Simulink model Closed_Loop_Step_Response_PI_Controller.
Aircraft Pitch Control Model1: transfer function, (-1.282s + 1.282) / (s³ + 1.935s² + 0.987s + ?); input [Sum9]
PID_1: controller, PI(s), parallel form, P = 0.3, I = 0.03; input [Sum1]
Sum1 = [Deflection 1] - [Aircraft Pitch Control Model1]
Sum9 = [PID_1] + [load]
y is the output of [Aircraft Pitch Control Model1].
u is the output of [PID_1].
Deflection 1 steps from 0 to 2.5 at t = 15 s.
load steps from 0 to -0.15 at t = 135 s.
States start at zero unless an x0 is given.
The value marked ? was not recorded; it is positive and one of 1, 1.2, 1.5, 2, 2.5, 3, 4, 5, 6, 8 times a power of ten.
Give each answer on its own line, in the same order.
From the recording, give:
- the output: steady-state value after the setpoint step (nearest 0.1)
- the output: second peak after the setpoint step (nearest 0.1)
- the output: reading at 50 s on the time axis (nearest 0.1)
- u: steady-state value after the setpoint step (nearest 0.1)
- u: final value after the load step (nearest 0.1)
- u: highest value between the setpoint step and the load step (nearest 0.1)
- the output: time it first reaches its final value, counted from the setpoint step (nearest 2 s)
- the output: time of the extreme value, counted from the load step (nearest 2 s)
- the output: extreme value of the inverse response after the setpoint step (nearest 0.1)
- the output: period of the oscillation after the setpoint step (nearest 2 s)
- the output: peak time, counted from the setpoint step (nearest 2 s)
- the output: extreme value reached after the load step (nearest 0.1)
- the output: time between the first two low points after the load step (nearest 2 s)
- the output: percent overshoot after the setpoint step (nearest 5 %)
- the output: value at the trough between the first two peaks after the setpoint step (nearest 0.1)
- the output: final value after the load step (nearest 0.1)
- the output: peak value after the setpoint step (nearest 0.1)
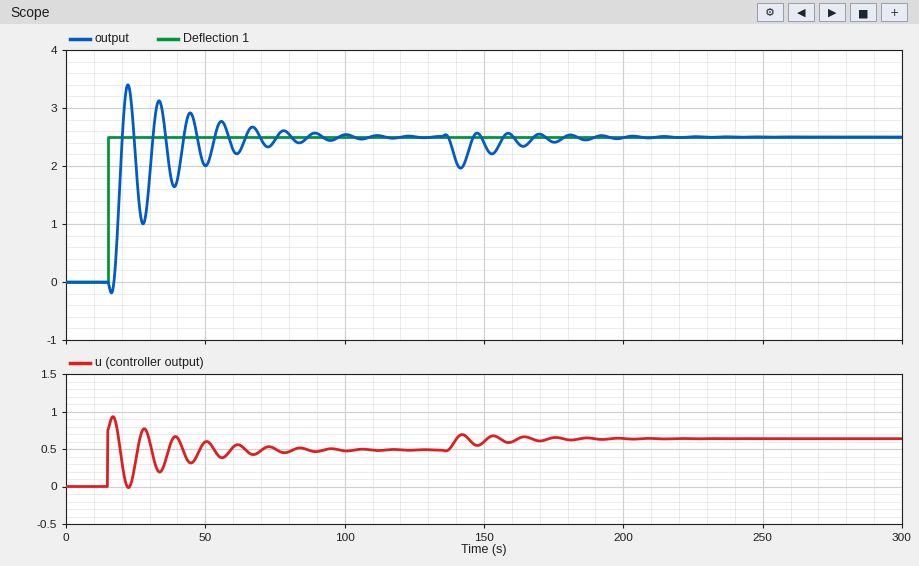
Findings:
2.5
3.1
2.0
0.5
0.6
0.9
6 s
6 s
-0.2
12 s
8 s
2.0
12 s
35 %
1.0
2.5
3.4
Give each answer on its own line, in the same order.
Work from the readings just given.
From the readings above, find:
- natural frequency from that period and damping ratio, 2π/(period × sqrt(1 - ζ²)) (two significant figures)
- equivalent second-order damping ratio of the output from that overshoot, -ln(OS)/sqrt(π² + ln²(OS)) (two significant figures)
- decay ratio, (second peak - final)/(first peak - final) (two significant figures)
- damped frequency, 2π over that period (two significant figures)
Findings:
0.55 rad/s
0.32
0.67
0.52 rad/s
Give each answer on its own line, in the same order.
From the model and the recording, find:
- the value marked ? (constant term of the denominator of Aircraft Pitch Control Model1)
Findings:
0.25
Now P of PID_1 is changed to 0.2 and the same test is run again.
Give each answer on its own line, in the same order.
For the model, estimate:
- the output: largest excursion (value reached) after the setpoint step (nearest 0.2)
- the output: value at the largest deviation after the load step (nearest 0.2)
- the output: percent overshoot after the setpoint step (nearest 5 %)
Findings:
2.8
2.0
15 %
